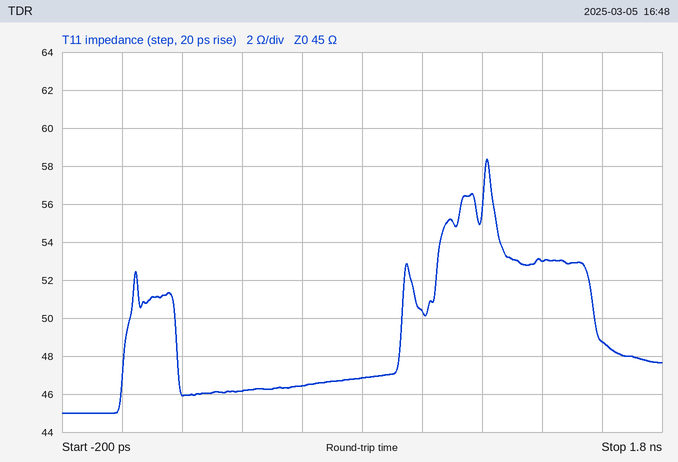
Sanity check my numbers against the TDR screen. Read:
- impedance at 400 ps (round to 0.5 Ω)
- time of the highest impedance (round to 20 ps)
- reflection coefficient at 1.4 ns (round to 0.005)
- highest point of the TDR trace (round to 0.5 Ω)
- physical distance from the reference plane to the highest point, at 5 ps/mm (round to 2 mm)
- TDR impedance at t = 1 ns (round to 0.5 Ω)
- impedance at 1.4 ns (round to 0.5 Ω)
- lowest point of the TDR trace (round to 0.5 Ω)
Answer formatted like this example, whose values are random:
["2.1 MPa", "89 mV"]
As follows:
["46.0 Ω", "1.22 ns", "+0.080", "58.5 Ω", "122 mm", "50.5 Ω", "53.0 Ω", "45.0 Ω"]
